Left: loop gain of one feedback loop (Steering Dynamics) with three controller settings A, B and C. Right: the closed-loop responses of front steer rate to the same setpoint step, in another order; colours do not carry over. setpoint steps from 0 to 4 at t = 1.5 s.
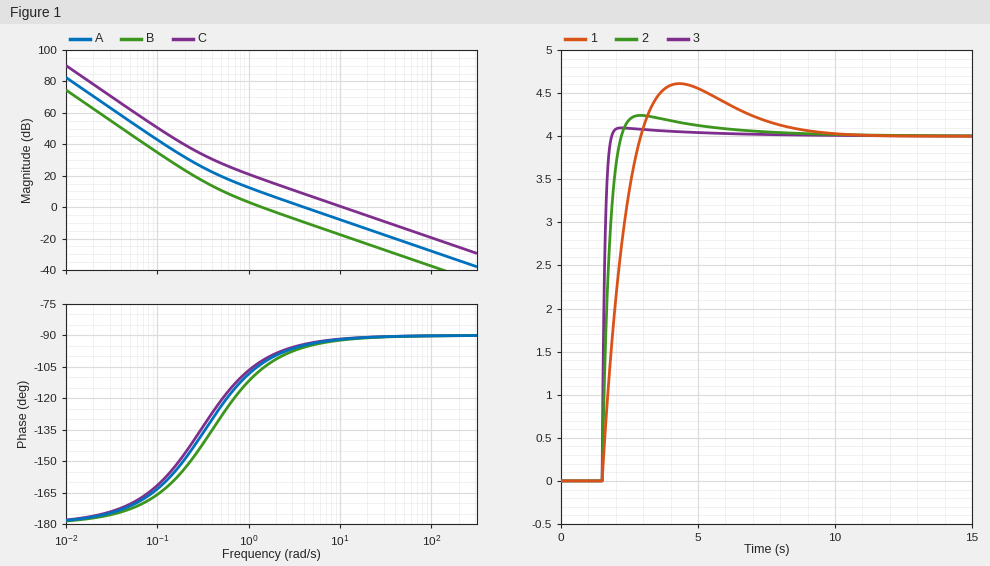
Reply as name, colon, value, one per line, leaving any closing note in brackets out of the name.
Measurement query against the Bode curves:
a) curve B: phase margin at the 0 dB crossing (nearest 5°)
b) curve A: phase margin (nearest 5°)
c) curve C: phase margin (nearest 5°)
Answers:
curve B: phase margin at the 0 dB crossing: 75°
curve A: phase margin: 85°
curve C: phase margin: 90°
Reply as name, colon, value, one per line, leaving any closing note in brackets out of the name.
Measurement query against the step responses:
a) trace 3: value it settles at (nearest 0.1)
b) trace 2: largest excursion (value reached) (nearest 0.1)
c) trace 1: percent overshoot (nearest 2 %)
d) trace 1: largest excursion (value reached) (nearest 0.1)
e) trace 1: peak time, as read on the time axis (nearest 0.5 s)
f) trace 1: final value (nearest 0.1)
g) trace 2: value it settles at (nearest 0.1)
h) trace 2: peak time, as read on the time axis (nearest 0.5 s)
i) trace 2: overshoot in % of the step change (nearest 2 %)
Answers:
trace 3: value it settles at: 4.0
trace 2: largest excursion (value reached): 4.2
trace 1: percent overshoot: 16 %
trace 1: largest excursion (value reached): 4.6
trace 1: peak time, as read on the time axis: 4.5 s
trace 1: final value: 4.0
trace 2: value it settles at: 4.0
trace 2: peak time, as read on the time axis: 3.0 s
trace 2: overshoot in % of the step change: 6 %
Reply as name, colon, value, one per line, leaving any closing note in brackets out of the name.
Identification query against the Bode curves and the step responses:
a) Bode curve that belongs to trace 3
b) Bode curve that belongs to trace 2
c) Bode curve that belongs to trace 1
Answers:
Bode curve that belongs to trace 3: C
Bode curve that belongs to trace 2: A
Bode curve that belongs to trace 1: B
